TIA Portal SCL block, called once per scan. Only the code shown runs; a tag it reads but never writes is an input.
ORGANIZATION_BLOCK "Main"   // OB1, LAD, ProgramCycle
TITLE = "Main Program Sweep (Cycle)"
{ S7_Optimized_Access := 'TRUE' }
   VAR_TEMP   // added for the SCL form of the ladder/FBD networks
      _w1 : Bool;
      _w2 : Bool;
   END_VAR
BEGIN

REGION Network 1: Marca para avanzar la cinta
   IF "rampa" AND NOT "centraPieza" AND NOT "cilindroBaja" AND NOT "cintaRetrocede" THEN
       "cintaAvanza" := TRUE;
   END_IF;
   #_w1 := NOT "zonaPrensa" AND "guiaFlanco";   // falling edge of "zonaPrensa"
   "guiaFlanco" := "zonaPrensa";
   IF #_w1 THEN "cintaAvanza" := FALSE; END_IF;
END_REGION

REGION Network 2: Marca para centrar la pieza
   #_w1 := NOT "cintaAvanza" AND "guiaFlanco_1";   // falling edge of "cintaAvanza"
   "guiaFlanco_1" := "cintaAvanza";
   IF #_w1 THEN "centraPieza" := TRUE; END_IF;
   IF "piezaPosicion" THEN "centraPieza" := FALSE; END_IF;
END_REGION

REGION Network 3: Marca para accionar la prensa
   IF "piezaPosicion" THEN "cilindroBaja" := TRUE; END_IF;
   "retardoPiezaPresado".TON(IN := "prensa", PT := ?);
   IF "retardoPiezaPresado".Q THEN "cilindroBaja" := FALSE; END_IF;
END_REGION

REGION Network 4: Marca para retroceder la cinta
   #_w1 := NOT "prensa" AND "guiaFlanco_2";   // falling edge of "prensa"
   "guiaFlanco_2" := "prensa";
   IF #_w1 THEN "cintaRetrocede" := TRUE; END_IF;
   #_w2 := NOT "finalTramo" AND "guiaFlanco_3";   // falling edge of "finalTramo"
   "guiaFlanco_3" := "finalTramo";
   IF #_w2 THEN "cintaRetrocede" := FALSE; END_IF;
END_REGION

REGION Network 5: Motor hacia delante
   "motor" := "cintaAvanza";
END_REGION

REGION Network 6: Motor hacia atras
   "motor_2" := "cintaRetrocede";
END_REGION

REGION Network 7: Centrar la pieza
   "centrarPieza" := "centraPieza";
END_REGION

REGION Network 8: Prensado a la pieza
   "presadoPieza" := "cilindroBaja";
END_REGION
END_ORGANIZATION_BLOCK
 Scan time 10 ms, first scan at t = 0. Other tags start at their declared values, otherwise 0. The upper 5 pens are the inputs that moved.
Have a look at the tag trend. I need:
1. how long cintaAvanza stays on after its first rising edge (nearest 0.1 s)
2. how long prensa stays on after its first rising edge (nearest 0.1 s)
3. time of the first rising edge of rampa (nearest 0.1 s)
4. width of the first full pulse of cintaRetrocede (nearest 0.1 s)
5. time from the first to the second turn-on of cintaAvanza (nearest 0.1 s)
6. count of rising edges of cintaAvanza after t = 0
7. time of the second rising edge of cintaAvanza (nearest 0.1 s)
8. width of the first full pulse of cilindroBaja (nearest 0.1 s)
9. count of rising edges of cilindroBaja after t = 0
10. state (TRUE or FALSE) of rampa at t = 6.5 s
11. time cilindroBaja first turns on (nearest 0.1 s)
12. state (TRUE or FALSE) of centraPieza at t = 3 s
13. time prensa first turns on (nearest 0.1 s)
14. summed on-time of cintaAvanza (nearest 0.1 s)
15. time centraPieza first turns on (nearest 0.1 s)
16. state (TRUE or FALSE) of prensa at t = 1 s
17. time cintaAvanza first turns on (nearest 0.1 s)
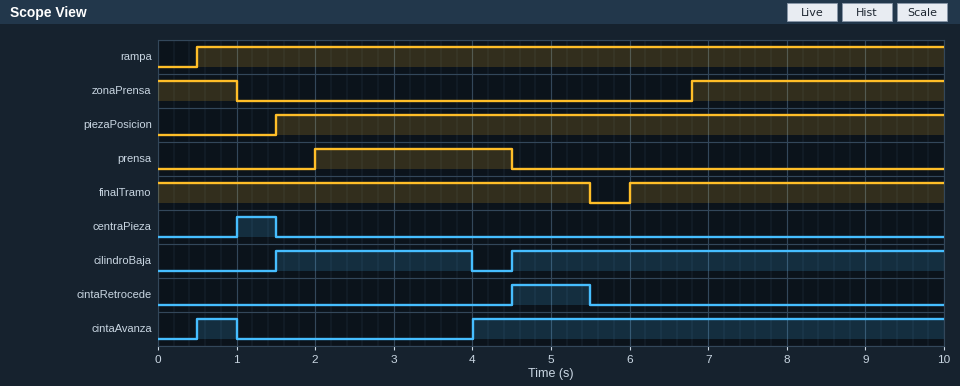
0.5 s
2.5 s
0.5 s
1.0 s
3.5 s
2
4.0 s
2.5 s
2
TRUE
1.5 s
FALSE
2.0 s
6.5 s
1.0 s
FALSE
0.5 s
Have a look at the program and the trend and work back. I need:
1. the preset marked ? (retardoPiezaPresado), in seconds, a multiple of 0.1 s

2.0 s
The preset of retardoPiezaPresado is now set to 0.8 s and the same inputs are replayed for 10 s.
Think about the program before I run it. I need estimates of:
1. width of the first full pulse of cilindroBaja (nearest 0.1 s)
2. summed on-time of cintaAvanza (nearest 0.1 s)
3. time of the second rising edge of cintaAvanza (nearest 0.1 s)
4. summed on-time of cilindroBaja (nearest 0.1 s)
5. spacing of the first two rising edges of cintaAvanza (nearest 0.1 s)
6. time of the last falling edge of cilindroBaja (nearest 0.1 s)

1.3 s
7.7 s
2.8 s
6.8 s
2.3 s
2.8 s
